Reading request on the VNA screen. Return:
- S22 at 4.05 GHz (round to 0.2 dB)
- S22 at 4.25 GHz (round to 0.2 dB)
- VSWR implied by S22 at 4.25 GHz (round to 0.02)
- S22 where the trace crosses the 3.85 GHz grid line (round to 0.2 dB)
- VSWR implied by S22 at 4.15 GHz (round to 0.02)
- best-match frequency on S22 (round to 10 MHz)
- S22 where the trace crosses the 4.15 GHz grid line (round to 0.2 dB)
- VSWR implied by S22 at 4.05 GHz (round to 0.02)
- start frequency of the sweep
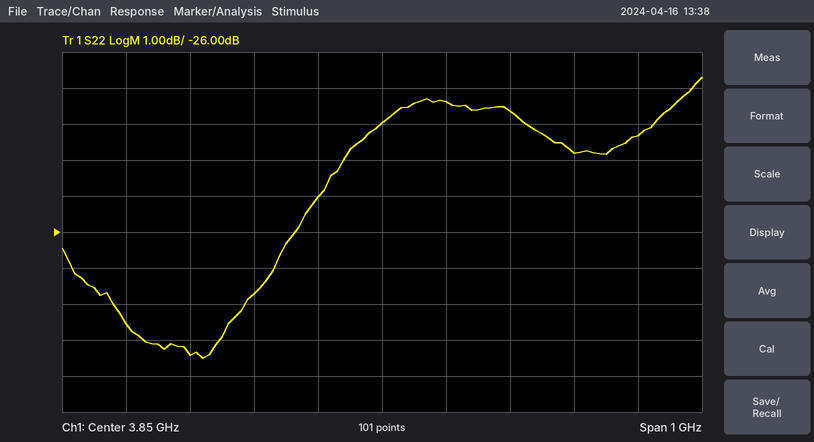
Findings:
-22.6 dB
-23.4 dB
1.14
-23.0 dB
1.14
3.57 GHz
-23.8 dB
1.16
3.35 GHz
